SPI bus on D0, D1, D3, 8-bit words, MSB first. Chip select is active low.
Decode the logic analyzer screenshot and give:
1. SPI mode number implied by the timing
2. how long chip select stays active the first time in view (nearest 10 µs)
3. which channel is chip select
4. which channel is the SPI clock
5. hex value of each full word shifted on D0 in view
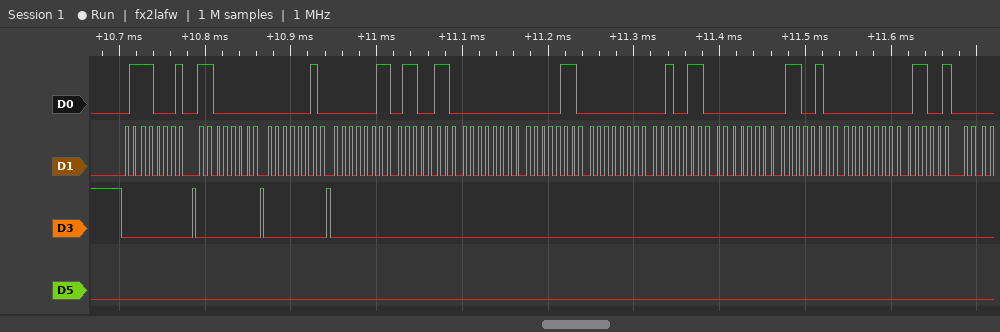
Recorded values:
0
80 µs
D3
D1
71, C0, 02, 03, 66, 00, 06, 00, 26, 00, 64, 00, 64
